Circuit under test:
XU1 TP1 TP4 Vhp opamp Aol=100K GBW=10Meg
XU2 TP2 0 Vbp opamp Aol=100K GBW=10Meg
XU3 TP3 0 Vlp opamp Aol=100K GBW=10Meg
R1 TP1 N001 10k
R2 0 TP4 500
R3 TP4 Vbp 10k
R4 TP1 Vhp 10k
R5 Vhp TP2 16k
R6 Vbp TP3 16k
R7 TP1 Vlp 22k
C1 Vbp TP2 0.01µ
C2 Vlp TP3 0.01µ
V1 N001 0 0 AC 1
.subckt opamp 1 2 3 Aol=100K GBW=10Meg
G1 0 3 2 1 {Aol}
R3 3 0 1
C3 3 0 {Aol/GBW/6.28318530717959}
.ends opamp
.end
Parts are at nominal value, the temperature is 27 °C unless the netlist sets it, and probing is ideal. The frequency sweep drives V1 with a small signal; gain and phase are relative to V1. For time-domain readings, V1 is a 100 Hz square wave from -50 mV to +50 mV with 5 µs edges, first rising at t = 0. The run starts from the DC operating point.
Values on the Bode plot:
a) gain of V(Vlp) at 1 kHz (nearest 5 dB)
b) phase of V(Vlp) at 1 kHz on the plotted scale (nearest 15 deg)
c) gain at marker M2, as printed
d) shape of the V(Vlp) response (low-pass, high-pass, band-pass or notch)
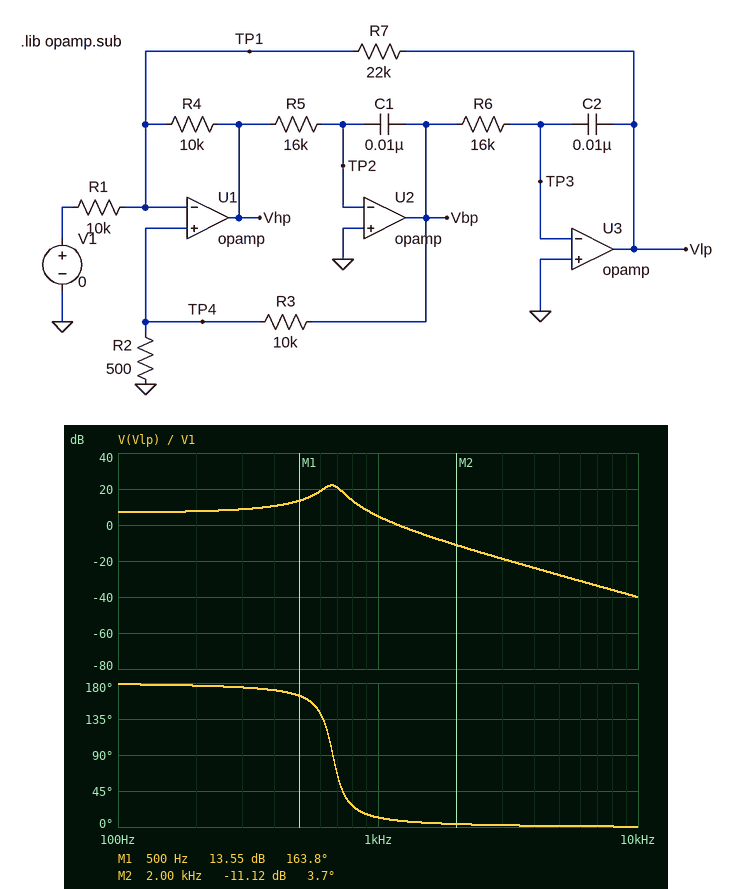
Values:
5 dB
15 deg
-11.12 dB
low-pass
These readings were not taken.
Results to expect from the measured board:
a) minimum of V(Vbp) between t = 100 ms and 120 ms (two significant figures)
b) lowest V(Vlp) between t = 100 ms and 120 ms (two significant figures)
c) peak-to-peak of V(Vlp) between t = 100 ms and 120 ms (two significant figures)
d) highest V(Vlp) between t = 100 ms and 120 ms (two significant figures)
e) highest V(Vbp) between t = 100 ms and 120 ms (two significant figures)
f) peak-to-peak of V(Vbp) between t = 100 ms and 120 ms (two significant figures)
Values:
-140 mV
-290 mV
580 mV
290 mV
140 mV
280 mV
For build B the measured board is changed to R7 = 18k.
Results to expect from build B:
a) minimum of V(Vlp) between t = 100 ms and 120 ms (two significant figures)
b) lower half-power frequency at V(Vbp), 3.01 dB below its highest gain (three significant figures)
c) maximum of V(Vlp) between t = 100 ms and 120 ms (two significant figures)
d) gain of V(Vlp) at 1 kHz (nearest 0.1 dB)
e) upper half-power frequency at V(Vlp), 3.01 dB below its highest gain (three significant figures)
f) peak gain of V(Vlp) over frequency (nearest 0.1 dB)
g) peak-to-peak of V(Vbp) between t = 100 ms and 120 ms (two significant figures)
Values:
-240 mV
683 Hz
240 mV
6.5 dB
795 Hz
20.9 dB
250 mV
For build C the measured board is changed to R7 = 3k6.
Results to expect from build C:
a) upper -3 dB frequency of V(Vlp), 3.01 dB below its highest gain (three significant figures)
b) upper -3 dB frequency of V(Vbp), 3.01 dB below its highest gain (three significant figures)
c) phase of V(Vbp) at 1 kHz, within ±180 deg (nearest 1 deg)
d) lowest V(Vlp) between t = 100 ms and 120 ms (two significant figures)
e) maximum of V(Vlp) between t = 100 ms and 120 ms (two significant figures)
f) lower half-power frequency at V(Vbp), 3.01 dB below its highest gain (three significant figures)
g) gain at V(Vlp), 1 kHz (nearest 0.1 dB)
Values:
1.76 kHz
1.77 kHz
83 deg
-47 mV
47 mV
1.55 kHz
-5.0 dB
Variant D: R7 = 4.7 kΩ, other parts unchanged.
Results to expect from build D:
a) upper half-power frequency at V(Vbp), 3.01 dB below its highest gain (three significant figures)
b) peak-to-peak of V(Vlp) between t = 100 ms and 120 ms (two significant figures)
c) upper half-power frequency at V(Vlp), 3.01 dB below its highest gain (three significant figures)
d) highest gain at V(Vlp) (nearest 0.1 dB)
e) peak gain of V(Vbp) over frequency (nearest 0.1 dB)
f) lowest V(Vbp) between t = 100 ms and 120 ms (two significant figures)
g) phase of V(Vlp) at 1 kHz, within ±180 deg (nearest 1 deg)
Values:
1.55 kHz
120 mV
1.54 kHz
10.9 dB
14.2 dB
-61 mV
170 deg
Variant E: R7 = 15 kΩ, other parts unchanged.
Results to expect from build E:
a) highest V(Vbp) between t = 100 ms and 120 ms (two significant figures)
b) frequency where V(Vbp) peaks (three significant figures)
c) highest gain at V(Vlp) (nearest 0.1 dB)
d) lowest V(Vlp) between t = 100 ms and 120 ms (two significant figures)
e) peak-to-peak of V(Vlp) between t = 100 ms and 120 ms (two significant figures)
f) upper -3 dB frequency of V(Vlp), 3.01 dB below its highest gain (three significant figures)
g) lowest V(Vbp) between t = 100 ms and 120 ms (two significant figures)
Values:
96 mV
812 Hz
19.7 dB
-180 mV
360 mV
868 Hz
-96 mV
